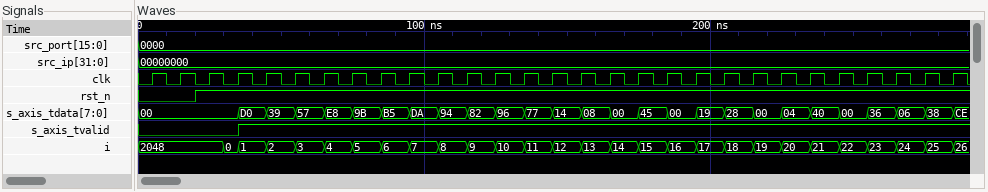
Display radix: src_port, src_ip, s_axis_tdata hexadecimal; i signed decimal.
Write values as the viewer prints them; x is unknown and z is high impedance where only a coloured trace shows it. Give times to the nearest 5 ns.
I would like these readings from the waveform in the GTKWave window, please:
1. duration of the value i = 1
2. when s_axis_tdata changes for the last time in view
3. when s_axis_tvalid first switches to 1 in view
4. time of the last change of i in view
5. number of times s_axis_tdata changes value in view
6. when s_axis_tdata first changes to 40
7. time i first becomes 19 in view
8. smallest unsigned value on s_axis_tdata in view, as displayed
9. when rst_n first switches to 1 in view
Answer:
10 ns
285 ns
35 ns
285 ns
26
235 ns
215 ns
00
20 ns
